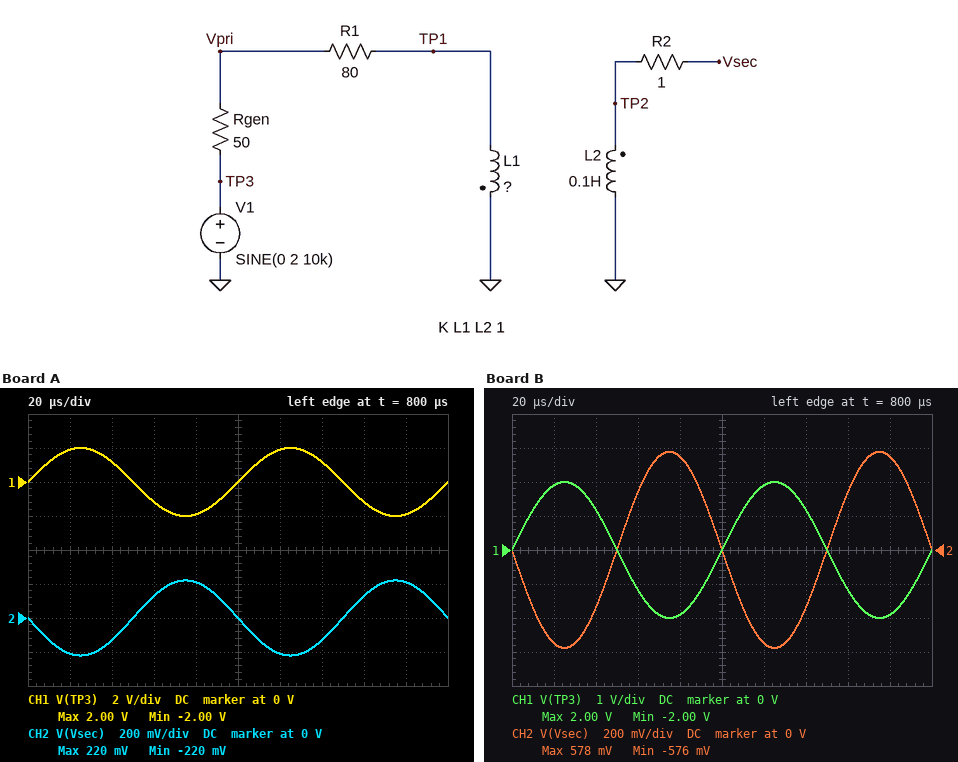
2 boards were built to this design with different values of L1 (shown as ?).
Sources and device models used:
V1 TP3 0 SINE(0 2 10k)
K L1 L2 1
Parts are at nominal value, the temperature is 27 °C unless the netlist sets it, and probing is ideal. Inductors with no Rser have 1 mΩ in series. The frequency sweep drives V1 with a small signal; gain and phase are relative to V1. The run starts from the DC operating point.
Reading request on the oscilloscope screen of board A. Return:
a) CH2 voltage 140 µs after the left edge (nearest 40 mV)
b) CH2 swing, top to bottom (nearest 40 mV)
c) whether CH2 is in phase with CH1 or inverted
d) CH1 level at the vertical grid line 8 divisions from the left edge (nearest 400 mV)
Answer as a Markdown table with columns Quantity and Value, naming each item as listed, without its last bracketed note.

| Quantity | Value |
|---|---|
| CH2 voltage 140 µs after the left edge | -120 mV |
| CH2 swing, top to bottom | 440 mV |
| whether CH2 is in phase with CH1 or inverted | inverted |
| CH1 level at the vertical grid line 8 divisions from the left edge | -1.2 V |
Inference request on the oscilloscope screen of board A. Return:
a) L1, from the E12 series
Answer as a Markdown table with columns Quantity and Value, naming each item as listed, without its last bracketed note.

| Quantity | Value |
|---|---|
| L1, from the E12 series | 8.2 H |
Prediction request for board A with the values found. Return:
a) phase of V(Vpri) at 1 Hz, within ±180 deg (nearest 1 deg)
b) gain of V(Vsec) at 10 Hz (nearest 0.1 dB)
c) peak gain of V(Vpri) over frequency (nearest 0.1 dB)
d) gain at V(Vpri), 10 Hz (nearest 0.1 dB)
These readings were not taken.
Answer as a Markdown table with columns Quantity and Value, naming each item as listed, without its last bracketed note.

| Quantity | Value |
|---|---|
| phase of V(Vpri) at 1 Hz, within ±180 deg | 11 deg |
| gain of V(Vsec) at 10 Hz | -19.4 dB |
| peak gain of V(Vpri) over frequency | 0 dB |
| gain at V(Vpri), 10 Hz | -0.2 dB |
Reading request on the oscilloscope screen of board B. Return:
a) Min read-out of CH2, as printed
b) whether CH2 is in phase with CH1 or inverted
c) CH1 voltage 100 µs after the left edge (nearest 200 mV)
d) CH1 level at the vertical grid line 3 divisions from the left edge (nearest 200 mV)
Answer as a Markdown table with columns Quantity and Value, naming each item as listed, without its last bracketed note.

| Quantity | Value |
|---|---|
| Min read-out of CH2, as printed | -576 mV |
| whether CH2 is in phase with CH1 or inverted | inverted |
| CH1 voltage 100 µs after the left edge | 0 V |
| CH1 level at the vertical grid line 3 divisions from the left edge | -1.2 V |
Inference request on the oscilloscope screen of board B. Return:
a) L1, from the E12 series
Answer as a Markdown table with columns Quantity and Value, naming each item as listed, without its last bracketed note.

| Quantity | Value |
|---|---|
| L1, from the E12 series | 1.2 H |
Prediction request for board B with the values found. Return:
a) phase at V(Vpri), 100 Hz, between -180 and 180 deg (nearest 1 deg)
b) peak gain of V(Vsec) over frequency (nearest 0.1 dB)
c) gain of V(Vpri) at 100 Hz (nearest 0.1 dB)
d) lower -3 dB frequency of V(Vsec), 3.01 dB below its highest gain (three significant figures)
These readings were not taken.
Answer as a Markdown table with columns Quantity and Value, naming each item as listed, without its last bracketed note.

| Quantity | Value |
|---|---|
| phase at V(Vpri), 100 Hz, between -180 and 180 deg | 4 deg |
| peak gain of V(Vsec) over frequency | -10.8 dB |
| gain of V(Vpri) at 100 Hz | -0.1 dB |
| lower -3 dB frequency of V(Vsec), 3.01 dB below its highest gain | 17.2 Hz |
